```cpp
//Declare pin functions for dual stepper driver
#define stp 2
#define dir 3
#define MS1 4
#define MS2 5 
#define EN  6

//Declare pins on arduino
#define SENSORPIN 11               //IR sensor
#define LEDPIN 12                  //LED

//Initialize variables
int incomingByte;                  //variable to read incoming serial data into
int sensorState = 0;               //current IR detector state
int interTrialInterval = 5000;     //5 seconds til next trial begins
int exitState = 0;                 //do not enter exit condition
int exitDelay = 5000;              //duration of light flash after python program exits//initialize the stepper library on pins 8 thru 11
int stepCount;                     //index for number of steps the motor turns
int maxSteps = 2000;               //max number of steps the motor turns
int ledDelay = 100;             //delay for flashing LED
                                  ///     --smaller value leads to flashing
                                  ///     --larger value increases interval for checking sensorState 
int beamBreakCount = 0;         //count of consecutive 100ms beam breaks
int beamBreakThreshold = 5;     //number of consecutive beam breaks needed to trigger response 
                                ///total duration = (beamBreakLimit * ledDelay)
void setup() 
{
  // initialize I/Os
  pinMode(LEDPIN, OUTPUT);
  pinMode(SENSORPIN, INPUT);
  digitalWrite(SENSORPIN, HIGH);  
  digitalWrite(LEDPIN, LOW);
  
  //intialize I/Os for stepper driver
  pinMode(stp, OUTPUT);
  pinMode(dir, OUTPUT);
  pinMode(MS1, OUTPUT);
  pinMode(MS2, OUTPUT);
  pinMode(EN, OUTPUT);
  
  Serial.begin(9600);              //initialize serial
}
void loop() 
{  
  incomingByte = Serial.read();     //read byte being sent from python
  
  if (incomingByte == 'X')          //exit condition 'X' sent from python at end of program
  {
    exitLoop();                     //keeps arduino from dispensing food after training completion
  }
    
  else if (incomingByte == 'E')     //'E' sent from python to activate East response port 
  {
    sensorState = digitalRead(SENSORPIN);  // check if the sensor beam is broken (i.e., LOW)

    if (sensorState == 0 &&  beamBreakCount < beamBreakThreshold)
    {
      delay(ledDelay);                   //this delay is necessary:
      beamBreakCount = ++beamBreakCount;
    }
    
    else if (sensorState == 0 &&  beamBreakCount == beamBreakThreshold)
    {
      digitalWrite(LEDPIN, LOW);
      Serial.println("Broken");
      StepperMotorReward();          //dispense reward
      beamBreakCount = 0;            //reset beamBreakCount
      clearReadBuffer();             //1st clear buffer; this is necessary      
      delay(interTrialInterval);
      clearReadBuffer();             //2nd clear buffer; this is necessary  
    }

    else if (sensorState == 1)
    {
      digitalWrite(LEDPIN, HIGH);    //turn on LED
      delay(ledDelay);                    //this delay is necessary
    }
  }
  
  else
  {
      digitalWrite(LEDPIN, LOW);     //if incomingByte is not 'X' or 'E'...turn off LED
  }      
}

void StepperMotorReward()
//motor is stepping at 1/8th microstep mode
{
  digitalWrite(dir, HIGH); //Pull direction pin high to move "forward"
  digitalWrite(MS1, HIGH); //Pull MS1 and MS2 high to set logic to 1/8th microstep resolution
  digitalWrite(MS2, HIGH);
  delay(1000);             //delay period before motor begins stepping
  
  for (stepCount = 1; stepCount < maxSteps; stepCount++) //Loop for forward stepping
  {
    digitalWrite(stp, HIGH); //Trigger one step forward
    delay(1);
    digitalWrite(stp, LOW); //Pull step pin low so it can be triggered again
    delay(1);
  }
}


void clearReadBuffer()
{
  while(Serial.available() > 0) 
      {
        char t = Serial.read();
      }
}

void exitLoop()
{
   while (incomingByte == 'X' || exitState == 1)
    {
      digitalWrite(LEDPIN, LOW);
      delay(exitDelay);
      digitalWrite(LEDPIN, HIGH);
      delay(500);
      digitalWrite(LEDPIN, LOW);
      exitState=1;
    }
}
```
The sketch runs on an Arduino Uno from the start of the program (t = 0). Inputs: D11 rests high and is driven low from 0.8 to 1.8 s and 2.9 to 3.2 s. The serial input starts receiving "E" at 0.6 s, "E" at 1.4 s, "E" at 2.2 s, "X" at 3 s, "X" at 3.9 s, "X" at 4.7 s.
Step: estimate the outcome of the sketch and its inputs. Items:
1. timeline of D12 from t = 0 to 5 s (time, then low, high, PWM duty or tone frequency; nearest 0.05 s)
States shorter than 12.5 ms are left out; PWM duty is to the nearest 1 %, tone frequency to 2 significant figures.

0 s low; 0.6 s high; 0.7 s low; 2.2 s high; 2.3 s low
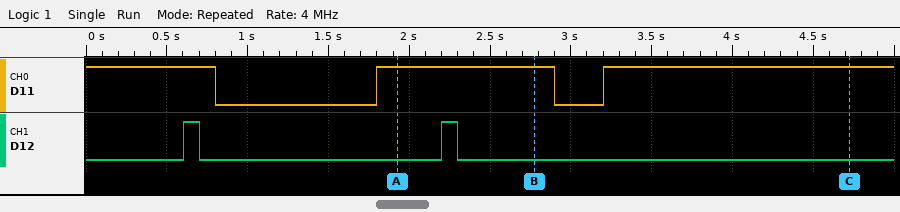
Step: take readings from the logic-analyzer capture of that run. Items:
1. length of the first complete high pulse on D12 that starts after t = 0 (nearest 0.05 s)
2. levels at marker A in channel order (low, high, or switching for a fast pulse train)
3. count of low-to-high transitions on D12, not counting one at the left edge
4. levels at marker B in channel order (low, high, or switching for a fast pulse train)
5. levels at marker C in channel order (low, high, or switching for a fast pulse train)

0.10 s
D11 high, D12 low
2
D11 high, D12 low
D11 high, D12 low
